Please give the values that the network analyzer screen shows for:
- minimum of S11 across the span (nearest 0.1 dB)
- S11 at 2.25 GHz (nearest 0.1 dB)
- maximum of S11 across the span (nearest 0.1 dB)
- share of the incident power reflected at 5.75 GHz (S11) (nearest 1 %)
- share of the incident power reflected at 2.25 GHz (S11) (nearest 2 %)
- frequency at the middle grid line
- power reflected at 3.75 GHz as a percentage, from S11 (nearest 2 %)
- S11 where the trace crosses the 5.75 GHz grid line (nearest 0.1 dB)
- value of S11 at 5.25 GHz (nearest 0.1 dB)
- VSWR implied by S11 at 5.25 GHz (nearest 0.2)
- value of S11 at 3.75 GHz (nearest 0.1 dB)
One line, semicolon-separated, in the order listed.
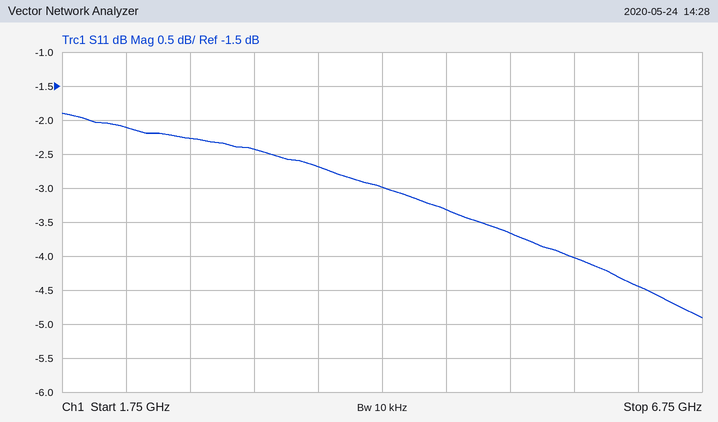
-4.9 dB; -2.1 dB; -1.9 dB; 40 %; 62 %; 4.25 GHz; 54 %; -4.0 dB; -3.7 dB; 4.8; -2.7 dB
